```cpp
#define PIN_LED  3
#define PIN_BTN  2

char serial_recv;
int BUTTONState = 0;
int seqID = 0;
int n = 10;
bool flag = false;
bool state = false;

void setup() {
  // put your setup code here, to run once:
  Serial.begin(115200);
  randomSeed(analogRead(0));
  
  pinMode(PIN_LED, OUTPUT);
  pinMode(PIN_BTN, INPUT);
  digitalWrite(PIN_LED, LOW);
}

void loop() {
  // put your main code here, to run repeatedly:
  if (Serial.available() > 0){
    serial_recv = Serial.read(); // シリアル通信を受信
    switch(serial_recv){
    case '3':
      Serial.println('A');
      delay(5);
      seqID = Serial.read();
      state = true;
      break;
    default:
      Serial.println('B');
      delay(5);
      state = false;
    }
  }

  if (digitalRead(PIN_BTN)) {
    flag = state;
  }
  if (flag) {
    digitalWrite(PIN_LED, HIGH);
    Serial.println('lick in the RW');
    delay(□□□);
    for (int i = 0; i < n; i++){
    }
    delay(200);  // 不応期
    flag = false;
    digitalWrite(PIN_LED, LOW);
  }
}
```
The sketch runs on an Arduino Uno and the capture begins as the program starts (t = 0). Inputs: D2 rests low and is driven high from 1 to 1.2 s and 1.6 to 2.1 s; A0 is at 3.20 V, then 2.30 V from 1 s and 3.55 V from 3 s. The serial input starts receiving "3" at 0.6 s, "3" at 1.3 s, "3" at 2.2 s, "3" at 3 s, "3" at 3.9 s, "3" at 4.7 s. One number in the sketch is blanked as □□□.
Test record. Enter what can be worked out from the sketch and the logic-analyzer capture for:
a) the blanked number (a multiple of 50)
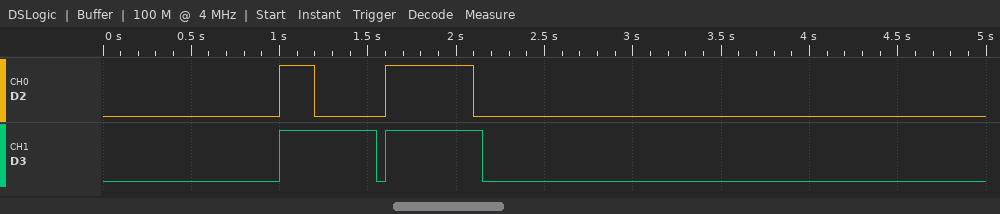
350
